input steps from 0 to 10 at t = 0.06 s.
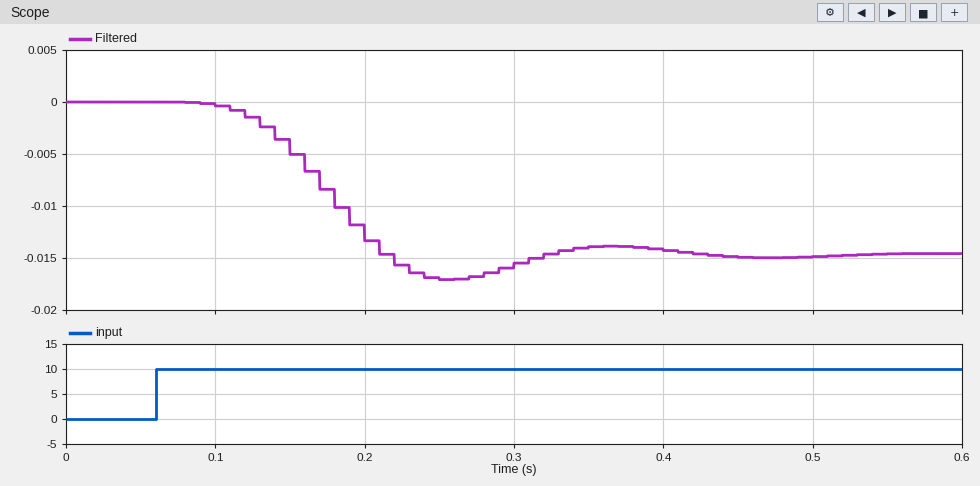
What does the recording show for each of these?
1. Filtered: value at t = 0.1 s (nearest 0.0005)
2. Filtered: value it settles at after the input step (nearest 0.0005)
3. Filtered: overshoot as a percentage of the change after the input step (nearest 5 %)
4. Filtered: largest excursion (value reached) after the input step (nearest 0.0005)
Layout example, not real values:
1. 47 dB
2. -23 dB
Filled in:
1. -0.0005
2. -0.0145
3. 15 %
4. -0.0170
